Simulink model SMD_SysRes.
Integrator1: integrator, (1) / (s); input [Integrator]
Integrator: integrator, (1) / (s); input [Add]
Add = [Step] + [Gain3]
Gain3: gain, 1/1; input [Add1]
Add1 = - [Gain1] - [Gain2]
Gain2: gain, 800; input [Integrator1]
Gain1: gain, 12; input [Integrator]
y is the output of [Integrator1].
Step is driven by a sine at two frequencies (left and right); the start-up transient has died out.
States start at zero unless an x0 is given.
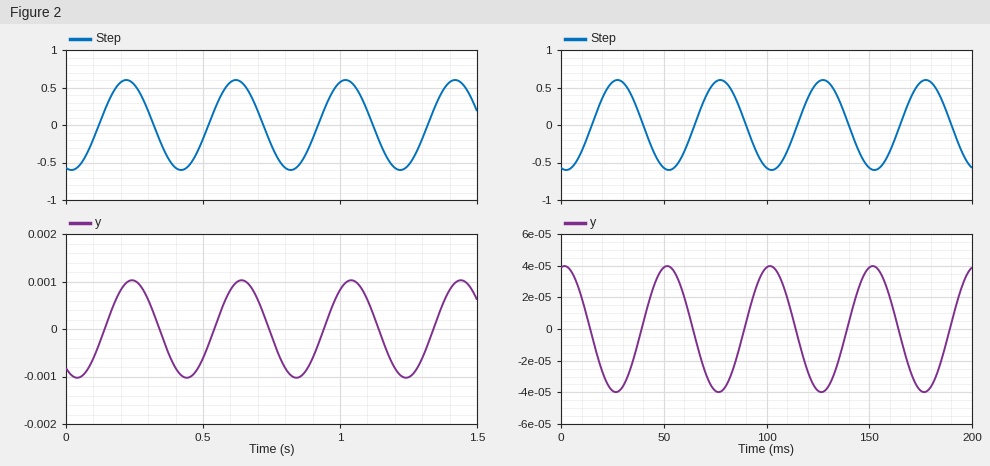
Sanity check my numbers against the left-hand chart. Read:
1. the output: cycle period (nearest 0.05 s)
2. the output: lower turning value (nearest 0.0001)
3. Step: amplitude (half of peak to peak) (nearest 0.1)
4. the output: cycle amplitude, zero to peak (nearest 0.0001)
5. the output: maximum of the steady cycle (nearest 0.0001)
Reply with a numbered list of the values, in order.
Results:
1. 0.40 s
2. -0.0010
3. 0.6
4. 0.0010
5. 0.0010
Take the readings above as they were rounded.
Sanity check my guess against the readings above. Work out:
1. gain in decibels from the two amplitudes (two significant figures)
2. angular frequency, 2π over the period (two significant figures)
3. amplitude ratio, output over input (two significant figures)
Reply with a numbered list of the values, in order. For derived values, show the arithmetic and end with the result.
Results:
1. 20 log10(0.001 / 0.6) = -56 dB
2. 2π / 0.4 = 16 rad/s
3. 0.001 / 0.6 = 0.0017
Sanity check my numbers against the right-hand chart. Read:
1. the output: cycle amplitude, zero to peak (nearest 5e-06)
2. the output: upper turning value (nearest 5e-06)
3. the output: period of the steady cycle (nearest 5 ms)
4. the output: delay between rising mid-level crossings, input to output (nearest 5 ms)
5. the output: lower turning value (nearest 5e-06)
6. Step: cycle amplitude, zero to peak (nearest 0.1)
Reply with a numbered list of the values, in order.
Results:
1. 0.000040
2. 0.000040
3. 50 ms
4. 25 ms
5. -0.000040
6. 0.6
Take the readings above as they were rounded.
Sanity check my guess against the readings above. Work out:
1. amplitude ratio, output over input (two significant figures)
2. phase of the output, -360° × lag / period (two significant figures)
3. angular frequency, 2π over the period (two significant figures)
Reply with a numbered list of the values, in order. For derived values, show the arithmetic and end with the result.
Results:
1. 4e-05 / 0.6 = 0.000067
2. -360 × 25 / 50 = -180°
3. 2π / 50 = 0.13 rad/ms
